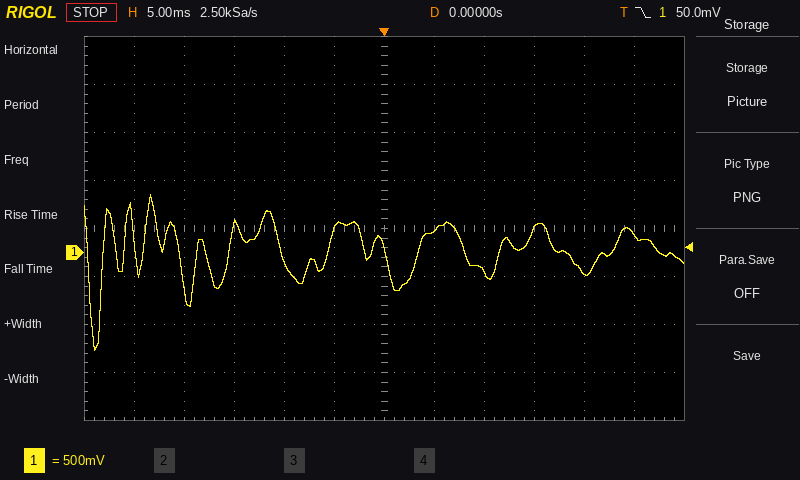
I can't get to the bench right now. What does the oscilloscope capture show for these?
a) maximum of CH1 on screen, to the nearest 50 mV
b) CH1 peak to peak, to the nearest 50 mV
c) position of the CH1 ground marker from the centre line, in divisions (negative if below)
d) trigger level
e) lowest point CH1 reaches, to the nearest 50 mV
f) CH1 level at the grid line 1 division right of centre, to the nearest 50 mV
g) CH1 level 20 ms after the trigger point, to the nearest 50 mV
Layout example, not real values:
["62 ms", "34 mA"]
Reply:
["600 mV", "1.60 V", "-0.5 div", "50.0 mV", "-1.00 V", "250 mV", "-200 mV"]
